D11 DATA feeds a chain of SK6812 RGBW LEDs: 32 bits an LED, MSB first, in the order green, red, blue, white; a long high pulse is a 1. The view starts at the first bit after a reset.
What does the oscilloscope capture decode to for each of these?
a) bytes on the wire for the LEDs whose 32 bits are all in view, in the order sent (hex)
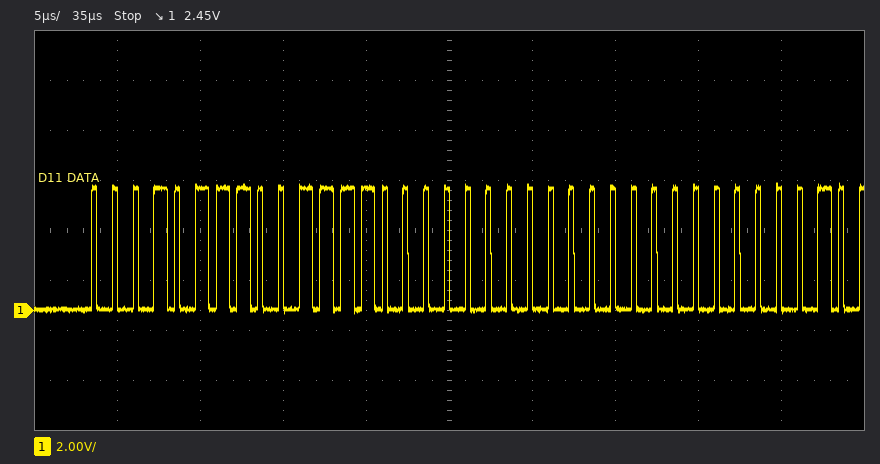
17 3C 00 00
